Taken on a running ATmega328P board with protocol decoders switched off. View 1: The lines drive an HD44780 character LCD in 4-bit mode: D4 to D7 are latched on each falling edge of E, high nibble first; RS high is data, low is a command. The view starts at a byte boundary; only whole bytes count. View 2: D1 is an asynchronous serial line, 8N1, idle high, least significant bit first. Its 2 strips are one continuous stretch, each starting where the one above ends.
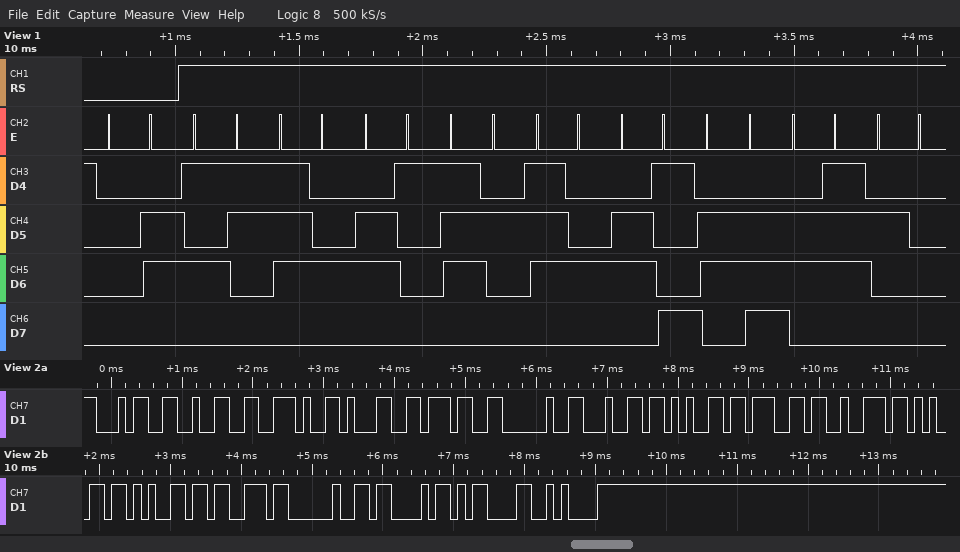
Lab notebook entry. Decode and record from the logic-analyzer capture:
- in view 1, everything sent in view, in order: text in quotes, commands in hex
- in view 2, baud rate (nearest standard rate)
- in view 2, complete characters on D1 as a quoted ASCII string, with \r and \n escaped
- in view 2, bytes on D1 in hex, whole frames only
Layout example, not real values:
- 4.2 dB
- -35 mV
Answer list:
- 0x06 "Starting "
- 9600 baud
- "42.17 degrees C\r\n"
- 34 32 2E 31 37 20 64 65 67 72 65 65 73 20 43 0D 0A
